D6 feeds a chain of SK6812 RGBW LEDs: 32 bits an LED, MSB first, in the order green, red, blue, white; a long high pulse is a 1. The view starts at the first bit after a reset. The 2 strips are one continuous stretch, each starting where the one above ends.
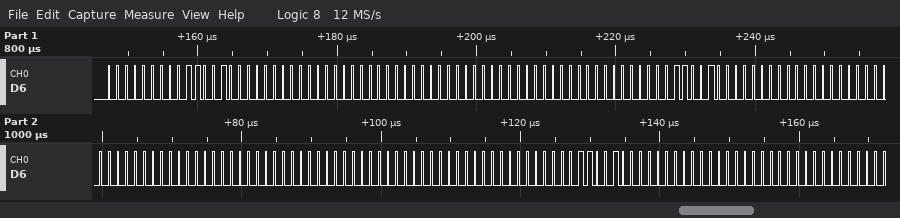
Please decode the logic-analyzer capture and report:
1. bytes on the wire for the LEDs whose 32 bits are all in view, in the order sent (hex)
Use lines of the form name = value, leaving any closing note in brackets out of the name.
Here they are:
bytes on the wire for the LEDs whose 32 bits are all in view, in the order sent = 00 64 00 00 00 00 00 00 64 00 00 00 00 00 00 00 00 00 64 00
